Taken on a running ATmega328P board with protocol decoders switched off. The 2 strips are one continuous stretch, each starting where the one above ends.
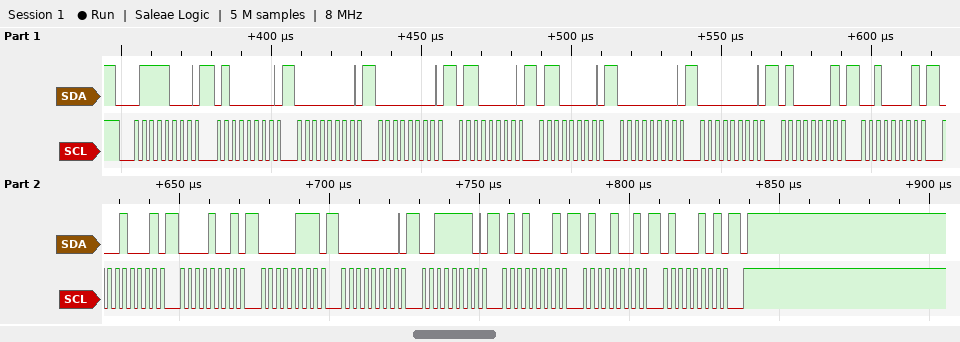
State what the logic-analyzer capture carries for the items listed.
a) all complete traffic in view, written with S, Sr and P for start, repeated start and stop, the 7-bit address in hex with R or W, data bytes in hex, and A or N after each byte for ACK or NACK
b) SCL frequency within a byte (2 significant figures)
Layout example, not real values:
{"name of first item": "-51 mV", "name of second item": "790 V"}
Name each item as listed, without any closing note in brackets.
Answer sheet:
{"all complete traffic in view, written with S, Sr and P for start, repeated start and stop, the 7-bit address in hex with R or W, data bytes in hex, and A or N after each byte for ACK or NACK": "S 3CW A 40 A 00 A 00 A 60 A 60 A 00 A 00 A 41 A 21 A 11 A 09 A 07 A 00 A 3E A 51 A 49 A 45 A P", "SCL frequency within a byte": "400 kHz"}
